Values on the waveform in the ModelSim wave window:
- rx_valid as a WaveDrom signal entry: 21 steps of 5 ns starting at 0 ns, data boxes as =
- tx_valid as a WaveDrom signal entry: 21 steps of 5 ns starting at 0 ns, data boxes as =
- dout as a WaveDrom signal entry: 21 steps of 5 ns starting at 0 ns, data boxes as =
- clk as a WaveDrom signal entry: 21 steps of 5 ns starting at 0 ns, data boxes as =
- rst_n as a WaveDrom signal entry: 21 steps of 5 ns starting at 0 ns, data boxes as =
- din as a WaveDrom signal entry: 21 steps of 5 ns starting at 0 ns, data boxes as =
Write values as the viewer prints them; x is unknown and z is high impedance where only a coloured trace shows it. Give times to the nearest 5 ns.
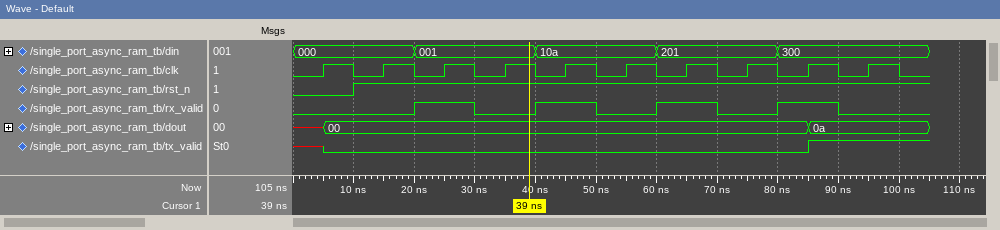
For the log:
{name: 'rx_valid', wave: '0...1.0.1.0.1.0.1.0..'}
{name: 'tx_valid', wave: 'x0...............1...'}
{name: 'dout', wave: 'x=...............=...', data: '00 0a'}
{name: 'clk', wave: '010101010101010101010'}
{name: 'rst_n', wave: '0.1..................'}
{name: 'din', wave: '=...=...=...=...=....', data: '000 001 10a 201 300'}
